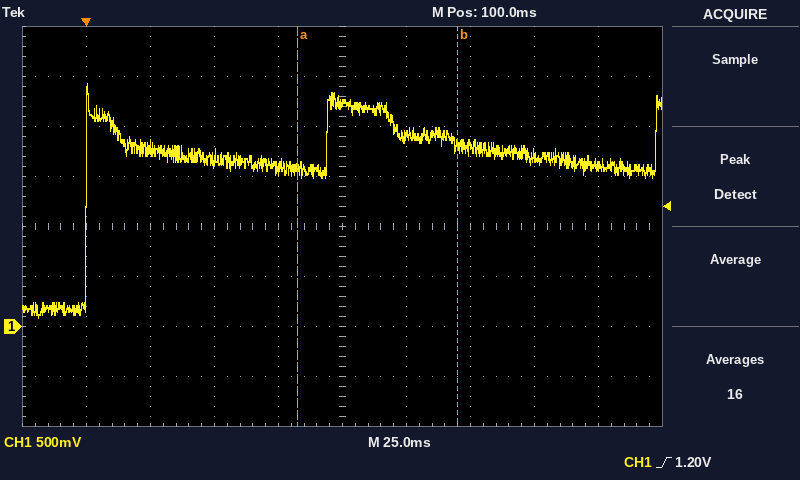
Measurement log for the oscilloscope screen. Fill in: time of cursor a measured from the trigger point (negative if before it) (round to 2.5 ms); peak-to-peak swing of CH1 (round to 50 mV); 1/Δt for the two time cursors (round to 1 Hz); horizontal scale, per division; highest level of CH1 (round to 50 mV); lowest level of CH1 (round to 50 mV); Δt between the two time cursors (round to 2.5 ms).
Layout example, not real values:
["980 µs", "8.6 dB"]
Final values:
["+82.5 ms", "2.35 V", "16 Hz", "25 ms", "2.45 V", "100 mV", "62.5 ms"]
